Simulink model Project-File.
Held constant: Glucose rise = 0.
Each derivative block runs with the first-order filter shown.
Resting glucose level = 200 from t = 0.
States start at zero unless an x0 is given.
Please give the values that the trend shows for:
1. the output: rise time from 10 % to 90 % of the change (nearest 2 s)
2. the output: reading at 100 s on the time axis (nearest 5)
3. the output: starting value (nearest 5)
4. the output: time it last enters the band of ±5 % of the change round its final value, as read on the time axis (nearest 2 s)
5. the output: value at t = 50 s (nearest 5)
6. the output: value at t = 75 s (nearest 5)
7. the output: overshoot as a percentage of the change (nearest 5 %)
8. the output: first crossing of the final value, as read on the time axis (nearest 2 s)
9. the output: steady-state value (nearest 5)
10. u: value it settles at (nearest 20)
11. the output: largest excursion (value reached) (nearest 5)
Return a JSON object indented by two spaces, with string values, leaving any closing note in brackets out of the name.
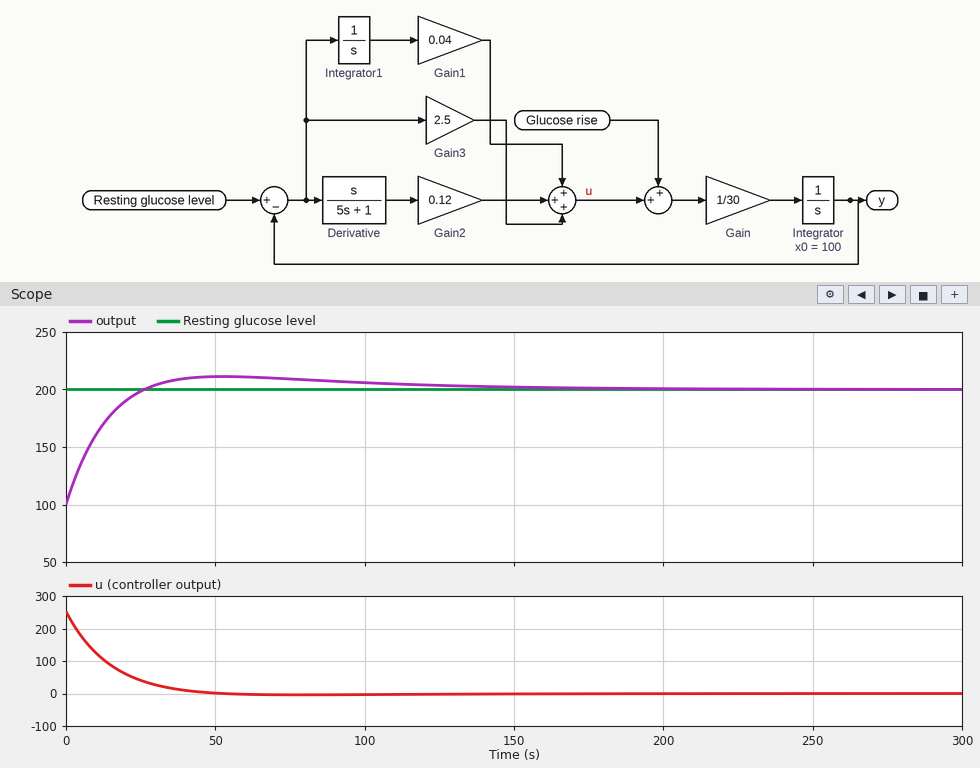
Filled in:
{
  "the output: rise time from 10 % to 90 % of the change": "18 s",
  "the output: reading at 100 s on the time axis": "205",
  "the output: starting value": "100",
  "the output: time it last enters the band of ±5 % of the change round its final value, as read on the time axis": "108 s",
  "the output: value at t = 50 s": "210",
  "the output: value at t = 75 s": "210",
  "the output: overshoot as a percentage of the change": "10 %",
  "the output: first crossing of the final value, as read on the time axis": "26 s",
  "the output: steady-state value": "200",
  "u: value it settles at": "0",
  "the output: largest excursion (value reached)": "210"
}
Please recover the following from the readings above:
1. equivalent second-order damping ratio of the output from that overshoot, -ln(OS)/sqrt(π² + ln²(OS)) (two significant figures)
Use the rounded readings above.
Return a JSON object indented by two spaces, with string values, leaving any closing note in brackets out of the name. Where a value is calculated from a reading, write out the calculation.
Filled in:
{
  "equivalent second-order damping ratio of the output from that overshoot, -ln(OS)/sqrt(π² + ln²(OS))": "ln(0.1) = -2.303; 2.303 / sqrt(9.870 + 5.302) = 0.59"
}
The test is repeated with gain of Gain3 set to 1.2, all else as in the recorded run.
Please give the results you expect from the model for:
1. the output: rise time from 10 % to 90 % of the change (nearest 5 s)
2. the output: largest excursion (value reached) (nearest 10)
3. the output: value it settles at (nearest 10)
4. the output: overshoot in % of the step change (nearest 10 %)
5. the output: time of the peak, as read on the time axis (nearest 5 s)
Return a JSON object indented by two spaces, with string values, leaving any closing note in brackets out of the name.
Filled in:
{
  "the output: rise time from 10 % to 90 % of the change": "25 s",
  "the output: largest excursion (value reached)": "230",
  "the output: value it settles at": "200",
  "the output: overshoot in % of the step change": "30 %",
  "the output: time of the peak, as read on the time axis": "65 s"
}
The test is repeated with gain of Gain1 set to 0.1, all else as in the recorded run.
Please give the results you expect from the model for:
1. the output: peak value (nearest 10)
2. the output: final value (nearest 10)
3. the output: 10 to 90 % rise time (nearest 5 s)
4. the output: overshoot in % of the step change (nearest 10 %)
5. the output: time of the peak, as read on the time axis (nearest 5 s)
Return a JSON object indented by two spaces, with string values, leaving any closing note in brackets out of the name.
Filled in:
{
  "the output: peak value": "220",
  "the output: final value": "200",
  "the output: 10 to 90 % rise time": "15 s",
  "the output: overshoot in % of the step change": "20 %",
  "the output: time of the peak, as read on the time axis": "40 s"
}
